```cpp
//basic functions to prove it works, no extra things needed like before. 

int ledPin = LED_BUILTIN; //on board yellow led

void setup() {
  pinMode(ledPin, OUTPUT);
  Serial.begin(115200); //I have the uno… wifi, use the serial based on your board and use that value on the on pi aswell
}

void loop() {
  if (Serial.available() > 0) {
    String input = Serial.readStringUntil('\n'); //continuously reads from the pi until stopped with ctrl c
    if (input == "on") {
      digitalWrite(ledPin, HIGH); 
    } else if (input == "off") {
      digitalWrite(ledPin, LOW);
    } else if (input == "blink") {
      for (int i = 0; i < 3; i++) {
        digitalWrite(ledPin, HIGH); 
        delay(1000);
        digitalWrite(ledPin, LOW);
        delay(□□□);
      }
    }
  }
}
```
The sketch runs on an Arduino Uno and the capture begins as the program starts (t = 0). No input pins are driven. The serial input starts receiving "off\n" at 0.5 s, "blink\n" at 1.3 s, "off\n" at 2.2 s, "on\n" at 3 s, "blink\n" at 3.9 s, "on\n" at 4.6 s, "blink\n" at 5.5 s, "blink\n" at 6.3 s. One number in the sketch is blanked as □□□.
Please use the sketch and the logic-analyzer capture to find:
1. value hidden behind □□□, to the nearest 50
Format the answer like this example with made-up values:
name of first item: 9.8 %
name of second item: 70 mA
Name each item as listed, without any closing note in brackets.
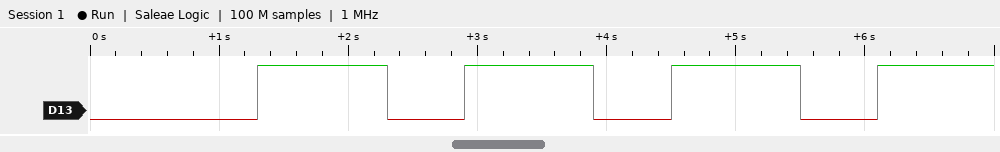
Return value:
value hidden behind □□□, to the nearest 50: 600
